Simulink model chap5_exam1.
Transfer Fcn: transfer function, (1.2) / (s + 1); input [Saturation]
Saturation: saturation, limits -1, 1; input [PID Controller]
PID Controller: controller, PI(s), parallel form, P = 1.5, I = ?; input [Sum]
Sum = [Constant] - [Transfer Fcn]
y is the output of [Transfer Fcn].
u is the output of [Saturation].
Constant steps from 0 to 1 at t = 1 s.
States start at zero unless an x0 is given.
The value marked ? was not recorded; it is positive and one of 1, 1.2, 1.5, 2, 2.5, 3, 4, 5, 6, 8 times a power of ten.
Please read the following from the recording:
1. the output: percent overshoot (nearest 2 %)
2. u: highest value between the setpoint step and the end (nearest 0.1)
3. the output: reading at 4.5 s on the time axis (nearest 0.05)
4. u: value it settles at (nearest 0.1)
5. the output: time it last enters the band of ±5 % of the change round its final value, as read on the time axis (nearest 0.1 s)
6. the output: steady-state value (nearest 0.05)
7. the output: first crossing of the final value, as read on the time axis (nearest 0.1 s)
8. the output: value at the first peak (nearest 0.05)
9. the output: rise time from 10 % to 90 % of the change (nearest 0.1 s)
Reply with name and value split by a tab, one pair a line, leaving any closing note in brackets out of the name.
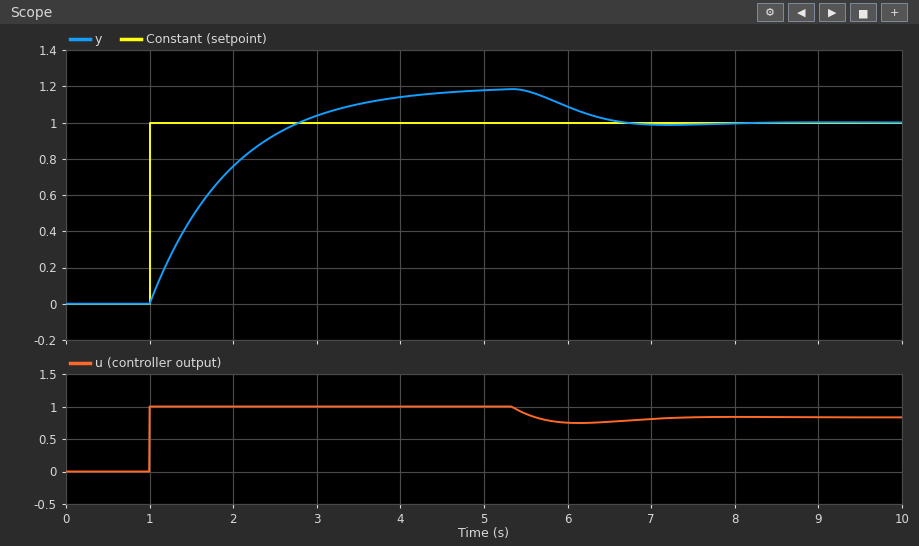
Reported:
the output: percent overshoot	18 %
u: highest value between the setpoint step and the end	1.0
the output: reading at 4.5 s on the time axis	1.15
u: value it settles at	0.8
the output: time it last enters the band of ±5 % of the change round its final value, as read on the time axis	6.2 s
the output: steady-state value	1.00
the output: first crossing of the final value, as read on the time axis	2.8 s
the output: value at the first peak	1.20
the output: rise time from 10 % to 90 % of the change	1.3 s
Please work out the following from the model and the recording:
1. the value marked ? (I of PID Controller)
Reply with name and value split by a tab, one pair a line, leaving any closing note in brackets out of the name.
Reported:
the value marked ?	4
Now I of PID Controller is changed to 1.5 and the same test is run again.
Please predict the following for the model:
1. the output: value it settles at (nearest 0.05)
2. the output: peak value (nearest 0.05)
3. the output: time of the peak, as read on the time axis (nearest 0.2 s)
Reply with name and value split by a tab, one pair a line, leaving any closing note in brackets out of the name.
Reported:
the output: value it settles at	1.00
the output: peak value	1.05
the output: time of the peak, as read on the time axis	3.6 s
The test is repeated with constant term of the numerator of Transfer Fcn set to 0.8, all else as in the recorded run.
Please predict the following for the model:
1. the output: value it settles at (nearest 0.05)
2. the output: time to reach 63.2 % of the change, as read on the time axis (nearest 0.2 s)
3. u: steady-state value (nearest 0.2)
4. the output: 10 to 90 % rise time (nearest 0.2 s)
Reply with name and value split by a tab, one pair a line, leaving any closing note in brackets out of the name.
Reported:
the output: value it settles at	0.80
the output: time to reach 63.2 % of the change, as read on the time axis	2.0 s
u: steady-state value	1.0
the output: 10 to 90 % rise time	2.2 s
